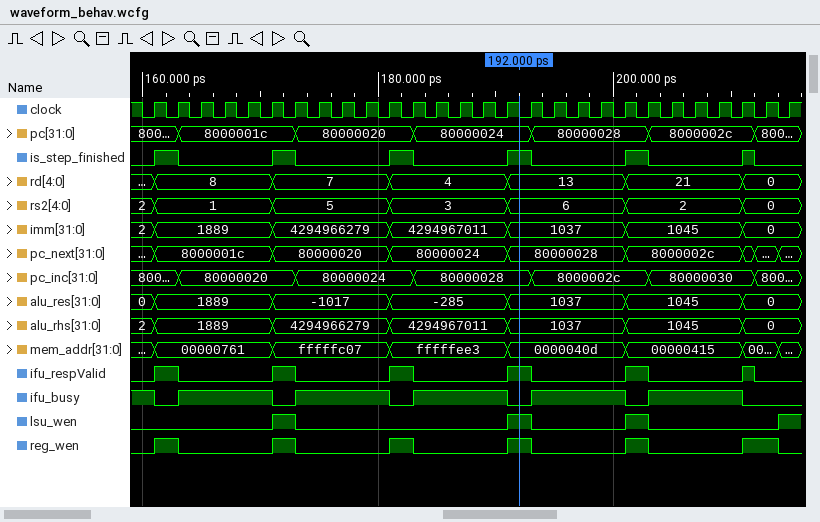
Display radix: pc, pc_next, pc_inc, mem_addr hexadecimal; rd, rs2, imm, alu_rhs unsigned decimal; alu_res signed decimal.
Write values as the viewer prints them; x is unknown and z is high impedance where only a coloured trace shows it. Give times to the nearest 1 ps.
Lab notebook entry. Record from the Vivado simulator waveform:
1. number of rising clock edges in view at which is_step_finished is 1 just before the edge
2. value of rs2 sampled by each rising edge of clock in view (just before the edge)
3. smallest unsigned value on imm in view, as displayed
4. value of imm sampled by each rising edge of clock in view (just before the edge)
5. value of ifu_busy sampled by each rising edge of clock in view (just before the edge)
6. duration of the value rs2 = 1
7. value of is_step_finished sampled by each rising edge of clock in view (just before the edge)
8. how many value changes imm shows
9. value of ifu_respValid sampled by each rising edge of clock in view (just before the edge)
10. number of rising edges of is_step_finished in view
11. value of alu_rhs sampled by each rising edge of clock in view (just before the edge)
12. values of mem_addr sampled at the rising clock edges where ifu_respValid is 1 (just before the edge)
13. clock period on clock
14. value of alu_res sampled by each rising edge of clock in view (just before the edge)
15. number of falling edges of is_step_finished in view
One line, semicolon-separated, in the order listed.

5; 2, 1, 1, 1, 1, 1, 5, 5, 5, 5, 5, 3, 3, 3, 3, 3, 6, 6, 6, 6, 6, 2, 2, 2, 2, 2, 0, 0; 0; 2, 1889, 1889, 1889, 1889, 1889, 4294966279, 4294966279, 4294966279, 4294966279, 4294966279, 4294967011, 4294967011, 4294967011, 4294967011, 4294967011, 1037, 1037, 1037, 1037, 1037, 1045, 1045, 1045, 1045, 1045, 0, 0; 1 0 1 1 1 1 0 1 1 1 1 0 1 1 1 1 0 1 1 1 1 0 1 1 1 1 0 0; 10 ps; 0 1 0 0 0 0 1 0 0 0 0 1 0 0 0 0 1 0 0 0 0 1 0 0 0 0 0 0; 6; 0 1 0 0 0 0 1 0 0 0 0 1 0 0 0 0 1 0 0 0 0 1 0 0 0 0 0 0; 6; 2, 1889, 1889, 1889, 1889, 1889, 4294966279, 4294966279, 4294966279, 4294966279, 4294966279, 4294967011, 4294967011, 4294967011, 4294967011, 4294967011, 1037, 1037, 1037, 1037, 1037, 1045, 1045, 1045, 1045, 1045, 0, 0; 00000761, fffffc07, fffffee3, 0000040d, 00000415; 2 ps; 0, 1889, 1889, 1889, 1889, 1889, -1017, -1017, -1017, -1017, -1017, -285, -285, -285, -285, -285, 1037, 1037, 1037, 1037, 1037, 1045, 1045, 1045, 1045, 1045, 0, 0; 6
